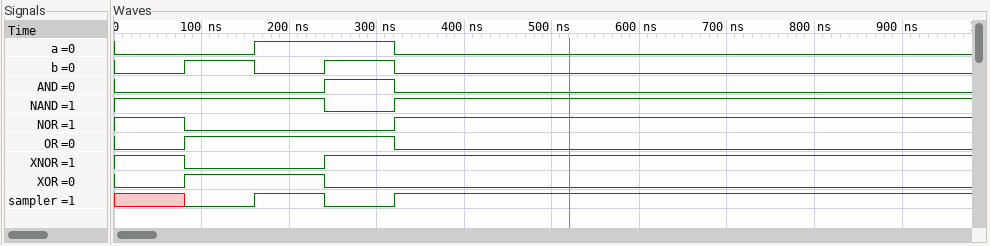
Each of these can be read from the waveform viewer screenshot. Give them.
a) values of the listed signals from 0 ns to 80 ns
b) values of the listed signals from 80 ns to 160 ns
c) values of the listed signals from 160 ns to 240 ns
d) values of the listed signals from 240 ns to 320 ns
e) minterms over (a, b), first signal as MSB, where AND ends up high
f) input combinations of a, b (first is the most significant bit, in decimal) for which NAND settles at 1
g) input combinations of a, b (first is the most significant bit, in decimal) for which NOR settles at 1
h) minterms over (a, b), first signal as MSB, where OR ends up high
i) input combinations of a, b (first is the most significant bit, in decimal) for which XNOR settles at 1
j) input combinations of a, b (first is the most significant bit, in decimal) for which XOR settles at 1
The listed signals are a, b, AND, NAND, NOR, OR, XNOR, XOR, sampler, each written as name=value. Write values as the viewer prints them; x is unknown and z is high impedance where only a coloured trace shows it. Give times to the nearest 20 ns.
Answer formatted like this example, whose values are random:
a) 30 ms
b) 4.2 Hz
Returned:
a) a=0, b=0, AND=0, NAND=1, NOR=1, OR=0, XNOR=1, XOR=0, sampler=x
b) a=0, b=1, AND=0, NAND=1, NOR=0, OR=1, XNOR=0, XOR=1, sampler=0
c) a=1, b=0, AND=0, NAND=1, NOR=0, OR=1, XNOR=0, XOR=1, sampler=1
d) a=1, b=1, AND=1, NAND=0, NOR=0, OR=1, XNOR=1, XOR=0, sampler=0
e) 3
f) 0, 1, 2
g) 0
h) 1, 2, 3
i) 0, 3
j) 1, 2
